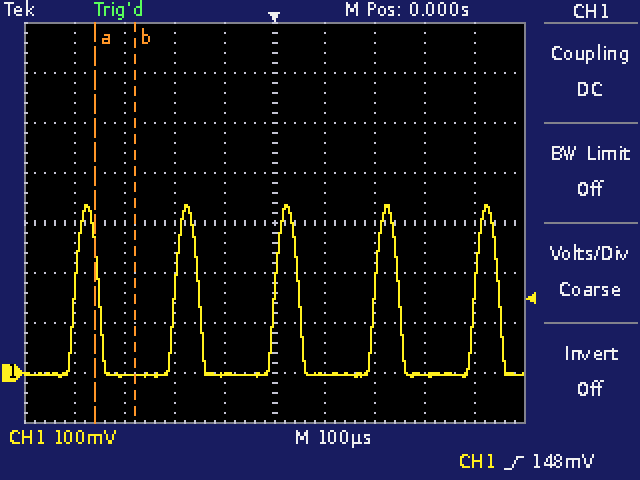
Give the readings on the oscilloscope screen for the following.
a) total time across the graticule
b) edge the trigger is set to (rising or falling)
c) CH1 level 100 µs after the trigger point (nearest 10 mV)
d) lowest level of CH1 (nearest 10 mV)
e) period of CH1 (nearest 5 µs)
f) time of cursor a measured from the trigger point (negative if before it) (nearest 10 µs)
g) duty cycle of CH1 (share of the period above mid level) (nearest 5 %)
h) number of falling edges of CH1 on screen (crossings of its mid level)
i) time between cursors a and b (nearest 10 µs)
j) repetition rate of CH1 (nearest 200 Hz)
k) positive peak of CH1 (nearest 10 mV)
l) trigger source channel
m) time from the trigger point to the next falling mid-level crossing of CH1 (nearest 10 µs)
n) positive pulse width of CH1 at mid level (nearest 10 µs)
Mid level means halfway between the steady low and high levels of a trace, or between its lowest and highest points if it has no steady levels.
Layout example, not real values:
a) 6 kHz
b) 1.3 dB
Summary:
a) 1 ms
b) rising
c) 0 mV
d) -10 mV
e) 200 µs
f) -360 µs
g) 25 %
h) 5
i) 80 µs
j) 5.0 kHz
k) 340 mV
l) CH1
m) 50 µs
n) 50 µs
